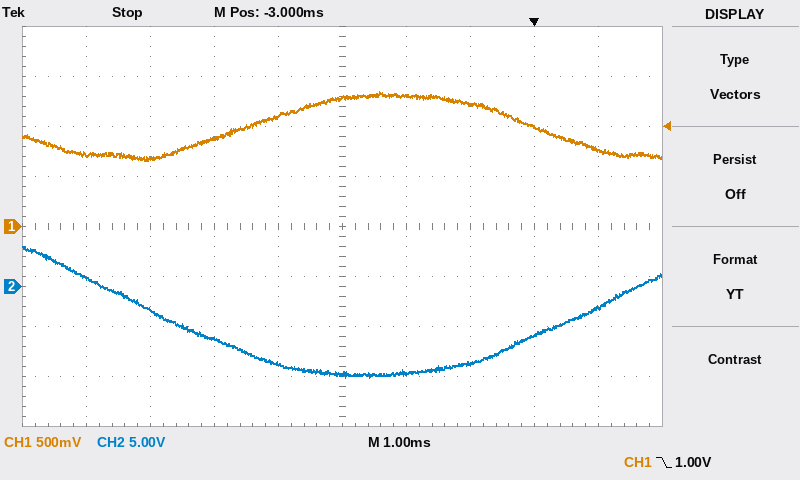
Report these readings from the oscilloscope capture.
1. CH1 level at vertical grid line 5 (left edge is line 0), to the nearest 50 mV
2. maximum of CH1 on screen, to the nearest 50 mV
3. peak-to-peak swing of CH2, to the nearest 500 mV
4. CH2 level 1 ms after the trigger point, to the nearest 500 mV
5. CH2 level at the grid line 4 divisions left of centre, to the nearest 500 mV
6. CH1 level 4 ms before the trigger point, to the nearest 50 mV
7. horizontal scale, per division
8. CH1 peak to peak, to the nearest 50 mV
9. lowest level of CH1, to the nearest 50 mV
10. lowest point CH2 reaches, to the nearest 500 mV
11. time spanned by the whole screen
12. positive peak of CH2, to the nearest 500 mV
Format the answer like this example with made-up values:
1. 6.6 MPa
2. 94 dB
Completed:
1. 1.30 V
2. 1.35 V
3. 13.0 V
4. -2.0 V
5. 1.0 V
6. 1.10 V
7. 1 ms
8. 700 mV
9. 650 mV
10. -9.0 V
11. 10 ms
12. 4.0 V
